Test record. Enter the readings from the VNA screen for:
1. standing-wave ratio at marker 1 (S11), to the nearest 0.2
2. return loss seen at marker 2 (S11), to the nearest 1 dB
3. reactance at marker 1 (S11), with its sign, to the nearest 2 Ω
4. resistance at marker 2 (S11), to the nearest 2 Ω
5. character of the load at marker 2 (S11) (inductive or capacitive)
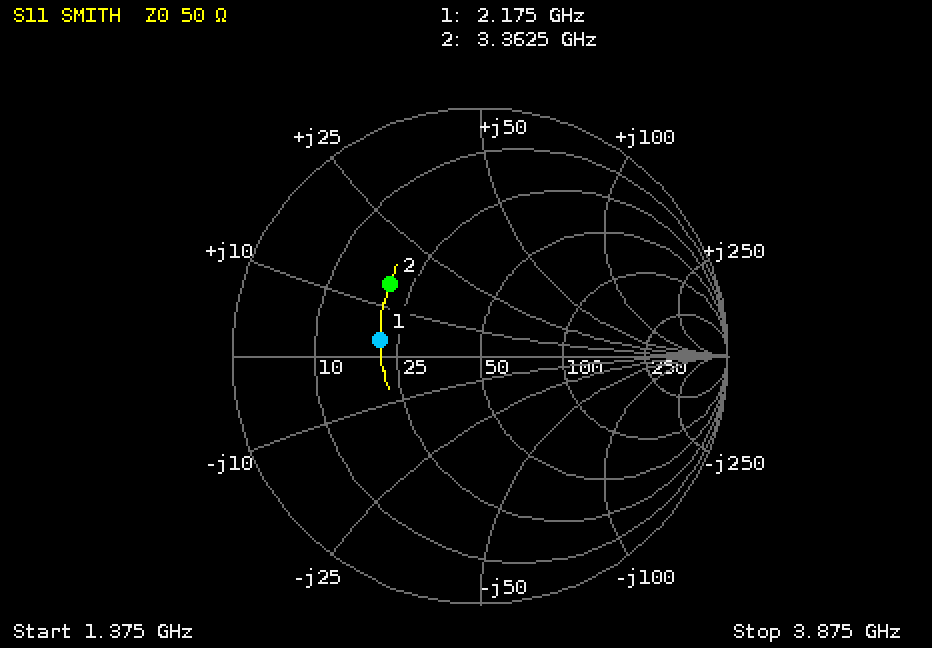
2.4
7 dB
+4 Ω
20 Ω
inductive
